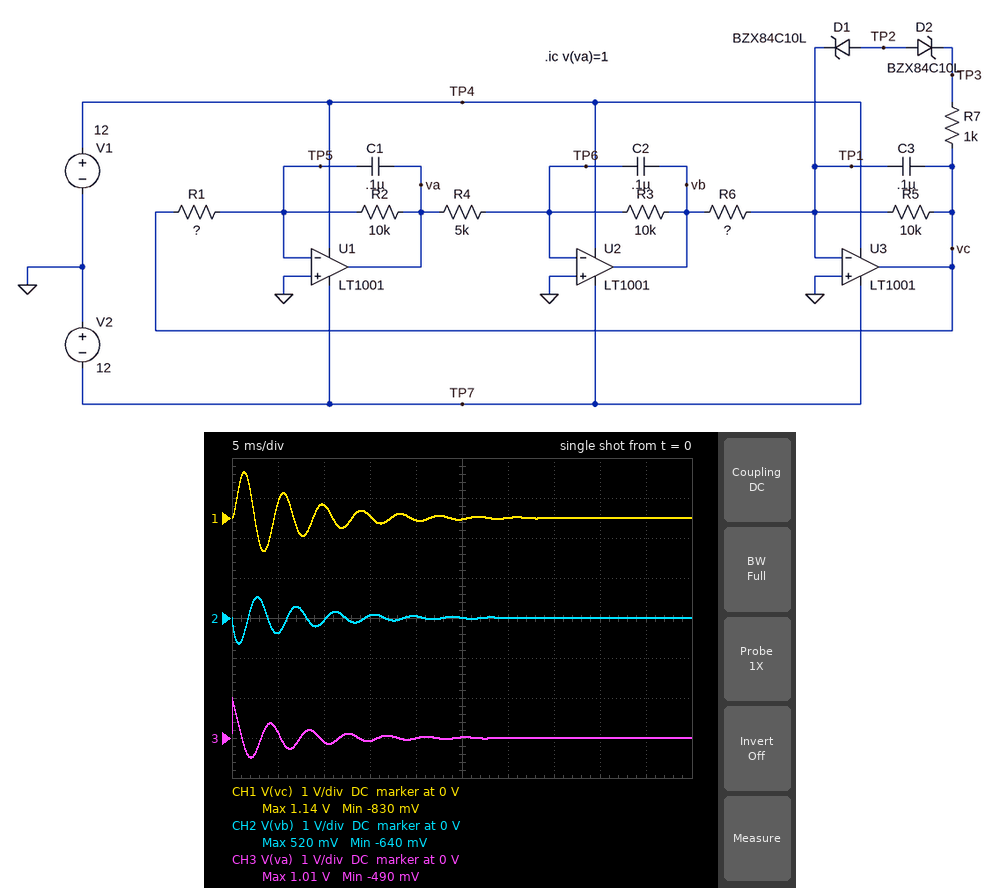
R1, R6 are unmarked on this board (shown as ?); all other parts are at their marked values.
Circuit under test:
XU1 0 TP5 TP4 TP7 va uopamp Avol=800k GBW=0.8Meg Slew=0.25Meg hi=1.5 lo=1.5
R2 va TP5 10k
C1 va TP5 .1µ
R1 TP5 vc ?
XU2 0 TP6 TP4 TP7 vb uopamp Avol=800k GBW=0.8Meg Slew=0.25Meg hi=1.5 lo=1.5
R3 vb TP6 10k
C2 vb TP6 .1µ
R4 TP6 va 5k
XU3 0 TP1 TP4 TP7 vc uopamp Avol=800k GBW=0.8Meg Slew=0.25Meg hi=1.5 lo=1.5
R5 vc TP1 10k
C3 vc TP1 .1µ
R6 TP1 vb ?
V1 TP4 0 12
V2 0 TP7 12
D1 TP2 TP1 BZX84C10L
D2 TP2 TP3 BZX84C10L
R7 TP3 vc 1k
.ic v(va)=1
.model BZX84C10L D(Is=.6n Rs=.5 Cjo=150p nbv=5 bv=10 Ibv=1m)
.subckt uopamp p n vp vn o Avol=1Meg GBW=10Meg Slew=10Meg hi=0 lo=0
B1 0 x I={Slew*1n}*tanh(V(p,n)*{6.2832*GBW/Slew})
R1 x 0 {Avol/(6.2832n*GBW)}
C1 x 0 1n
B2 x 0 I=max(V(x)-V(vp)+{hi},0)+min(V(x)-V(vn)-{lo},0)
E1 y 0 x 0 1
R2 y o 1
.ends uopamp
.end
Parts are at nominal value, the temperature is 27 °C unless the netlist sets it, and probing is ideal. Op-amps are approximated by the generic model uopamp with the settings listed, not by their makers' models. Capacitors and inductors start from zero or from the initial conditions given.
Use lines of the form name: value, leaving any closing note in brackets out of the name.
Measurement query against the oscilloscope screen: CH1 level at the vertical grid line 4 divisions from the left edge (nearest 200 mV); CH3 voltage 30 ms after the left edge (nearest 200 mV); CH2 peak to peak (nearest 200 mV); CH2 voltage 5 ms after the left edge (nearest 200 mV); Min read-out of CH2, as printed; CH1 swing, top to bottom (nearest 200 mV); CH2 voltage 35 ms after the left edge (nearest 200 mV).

CH1 level at the vertical grid line 4 divisions from the left edge: 0 V
CH3 voltage 30 ms after the left edge: 0 V
CH2 peak to peak: 1.2 V
CH2 voltage 5 ms after the left edge: -400 mV
Min read-out of CH2, as printed: -640 mV
CH1 swing, top to bottom: 2.0 V
CH2 voltage 35 ms after the left edge: 0 V
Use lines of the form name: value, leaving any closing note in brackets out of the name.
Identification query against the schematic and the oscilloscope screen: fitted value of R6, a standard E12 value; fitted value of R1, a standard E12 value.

fitted value of R6, a standard E12 value: 3.3 kΩ
fitted value of R1, a standard E12 value: 12 kΩ
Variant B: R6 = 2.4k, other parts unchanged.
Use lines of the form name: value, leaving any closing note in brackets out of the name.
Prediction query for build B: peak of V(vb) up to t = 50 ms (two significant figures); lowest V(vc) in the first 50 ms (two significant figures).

peak of V(vb) up to t = 50 ms: 620 mV
lowest V(vc) in the first 50 ms: -1.3 V
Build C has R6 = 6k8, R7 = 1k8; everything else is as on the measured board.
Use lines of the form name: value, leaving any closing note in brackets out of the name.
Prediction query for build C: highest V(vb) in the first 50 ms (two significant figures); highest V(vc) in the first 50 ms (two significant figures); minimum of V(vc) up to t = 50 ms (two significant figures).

highest V(vb) in the first 50 ms: 320 mV
highest V(vc) in the first 50 ms: 640 mV
minimum of V(vc) up to t = 50 ms: -260 mV
